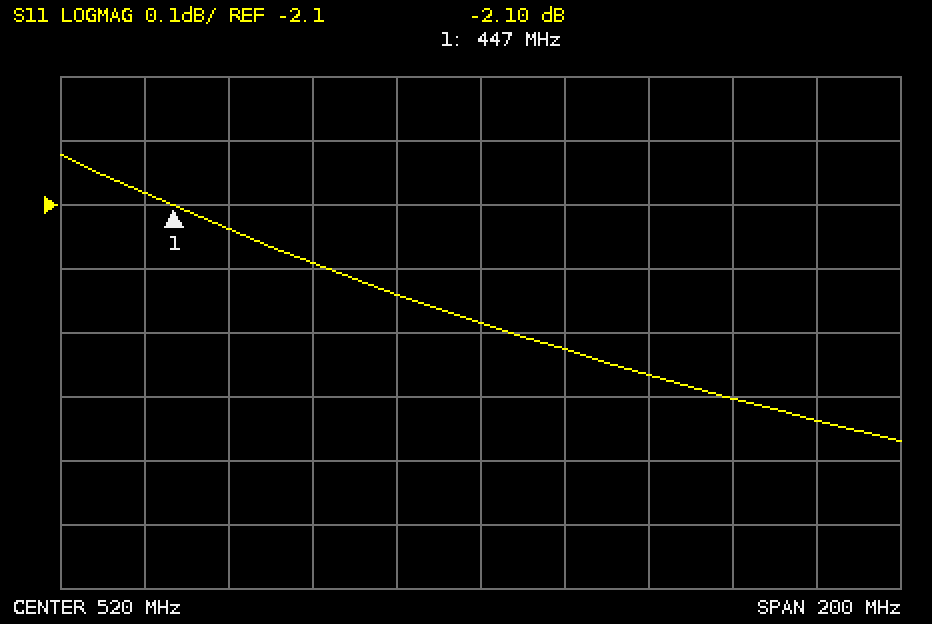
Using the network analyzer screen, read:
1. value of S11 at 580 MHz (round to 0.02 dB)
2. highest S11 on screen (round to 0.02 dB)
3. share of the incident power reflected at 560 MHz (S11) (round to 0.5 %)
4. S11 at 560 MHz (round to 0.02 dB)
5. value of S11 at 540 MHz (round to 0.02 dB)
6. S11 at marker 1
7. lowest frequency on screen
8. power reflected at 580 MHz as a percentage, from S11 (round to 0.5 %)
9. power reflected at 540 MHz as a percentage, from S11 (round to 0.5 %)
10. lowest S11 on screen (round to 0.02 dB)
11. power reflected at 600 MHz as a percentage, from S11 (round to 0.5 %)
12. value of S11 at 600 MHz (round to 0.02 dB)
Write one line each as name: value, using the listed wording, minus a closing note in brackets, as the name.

value of S11 at 580 MHz: -2.40 dB
highest S11 on screen: -2.02 dB
share of the incident power reflected at 560 MHz (S11): 58.0 %
S11 at 560 MHz: -2.36 dB
value of S11 at 540 MHz: -2.32 dB
S11 at marker 1: -2.10 dB
lowest frequency on screen: 420 MHz
power reflected at 580 MHz as a percentage, from S11: 57.5 %
power reflected at 540 MHz as a percentage, from S11: 58.5 %
lowest S11 on screen: -2.46 dB
power reflected at 600 MHz as a percentage, from S11: 57.0 %
value of S11 at 600 MHz: -2.44 dB
